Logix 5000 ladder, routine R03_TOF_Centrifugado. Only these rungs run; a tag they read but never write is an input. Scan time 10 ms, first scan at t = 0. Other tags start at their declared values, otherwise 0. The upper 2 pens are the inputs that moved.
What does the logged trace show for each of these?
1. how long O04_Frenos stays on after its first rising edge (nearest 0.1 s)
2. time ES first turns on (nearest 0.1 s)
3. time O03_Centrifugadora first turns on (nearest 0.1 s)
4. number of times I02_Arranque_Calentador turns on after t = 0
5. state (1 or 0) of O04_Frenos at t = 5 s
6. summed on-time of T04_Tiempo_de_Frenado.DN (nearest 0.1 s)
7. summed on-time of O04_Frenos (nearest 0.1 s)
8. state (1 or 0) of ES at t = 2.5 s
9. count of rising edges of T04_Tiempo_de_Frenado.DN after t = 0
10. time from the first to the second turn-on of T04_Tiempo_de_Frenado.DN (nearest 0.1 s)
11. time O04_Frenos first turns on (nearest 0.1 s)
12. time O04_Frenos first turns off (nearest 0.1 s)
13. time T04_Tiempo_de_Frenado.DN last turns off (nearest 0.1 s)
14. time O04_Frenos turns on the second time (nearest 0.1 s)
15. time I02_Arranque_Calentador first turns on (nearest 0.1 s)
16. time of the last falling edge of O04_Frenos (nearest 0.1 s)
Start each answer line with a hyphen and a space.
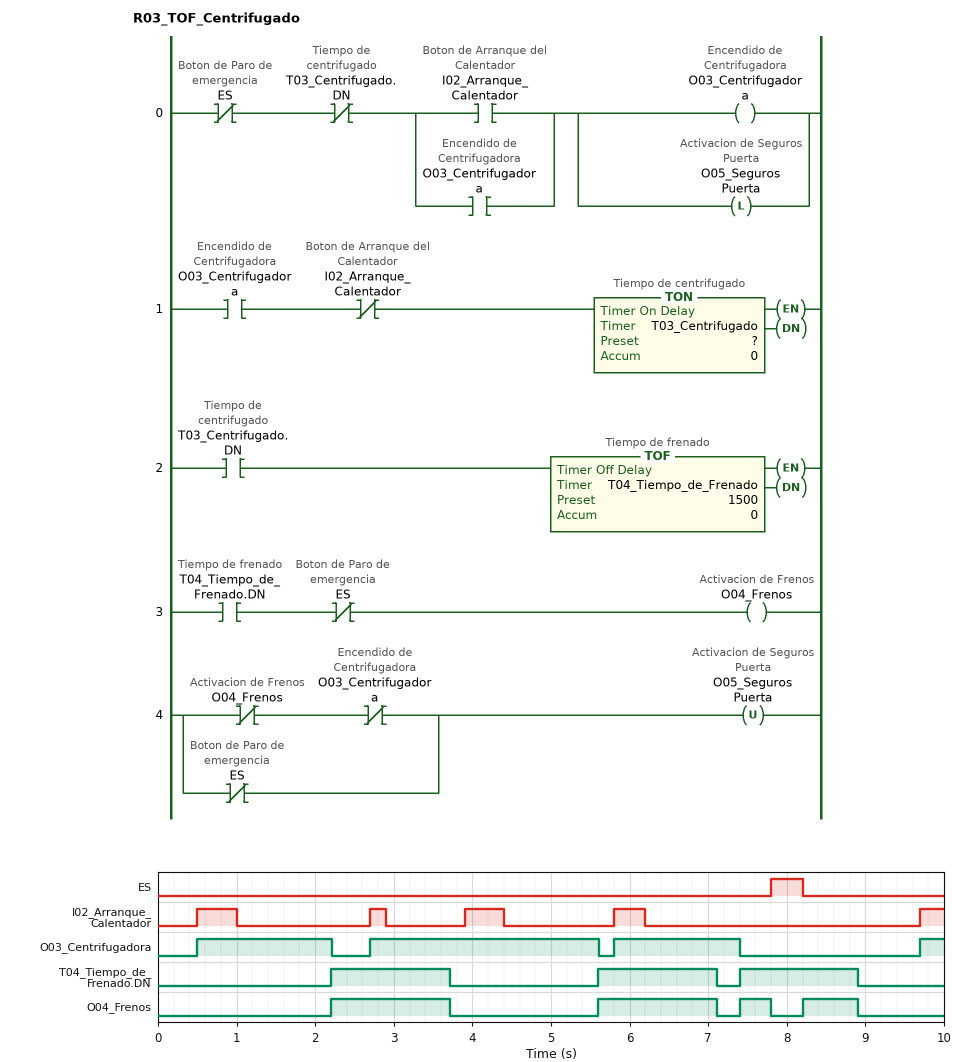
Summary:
- 1.5 s
- 7.8 s
- 0.5 s
- 5
- 0
- 4.5 s
- 4.1 s
- 0
- 3
- 3.4 s
- 2.2 s
- 3.7 s
- 8.9 s
- 5.6 s
- 0.5 s
- 8.9 s
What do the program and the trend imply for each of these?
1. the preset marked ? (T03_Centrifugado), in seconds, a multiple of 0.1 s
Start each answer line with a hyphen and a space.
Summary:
- 1.2 s
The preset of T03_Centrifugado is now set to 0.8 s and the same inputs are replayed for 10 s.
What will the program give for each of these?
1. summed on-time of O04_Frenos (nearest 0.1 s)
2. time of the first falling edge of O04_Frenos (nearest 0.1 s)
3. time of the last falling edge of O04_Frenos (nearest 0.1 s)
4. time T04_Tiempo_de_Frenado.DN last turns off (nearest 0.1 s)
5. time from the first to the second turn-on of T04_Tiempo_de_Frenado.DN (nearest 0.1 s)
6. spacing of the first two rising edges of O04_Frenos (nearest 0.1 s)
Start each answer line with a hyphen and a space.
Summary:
- 5.6 s
- 3.3 s
- 8.5 s
- 8.5 s
- 1.9 s
- 1.9 s
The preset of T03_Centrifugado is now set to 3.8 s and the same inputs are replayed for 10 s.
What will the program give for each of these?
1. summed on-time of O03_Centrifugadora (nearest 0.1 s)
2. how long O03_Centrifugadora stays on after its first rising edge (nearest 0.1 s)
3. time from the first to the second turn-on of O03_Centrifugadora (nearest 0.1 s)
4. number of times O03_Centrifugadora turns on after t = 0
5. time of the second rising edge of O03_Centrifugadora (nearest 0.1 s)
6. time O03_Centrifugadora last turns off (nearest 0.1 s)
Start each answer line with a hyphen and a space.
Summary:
- 7.6 s
- 7.3 s
- 9.2 s
- 2
- 9.7 s
- 7.8 s
